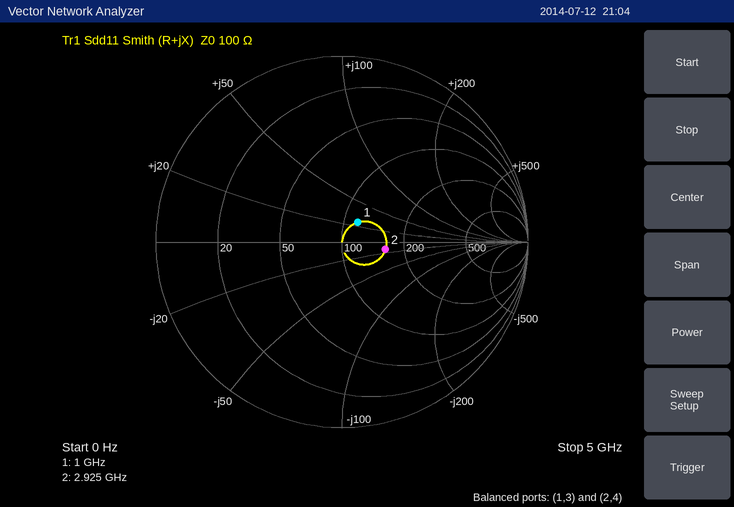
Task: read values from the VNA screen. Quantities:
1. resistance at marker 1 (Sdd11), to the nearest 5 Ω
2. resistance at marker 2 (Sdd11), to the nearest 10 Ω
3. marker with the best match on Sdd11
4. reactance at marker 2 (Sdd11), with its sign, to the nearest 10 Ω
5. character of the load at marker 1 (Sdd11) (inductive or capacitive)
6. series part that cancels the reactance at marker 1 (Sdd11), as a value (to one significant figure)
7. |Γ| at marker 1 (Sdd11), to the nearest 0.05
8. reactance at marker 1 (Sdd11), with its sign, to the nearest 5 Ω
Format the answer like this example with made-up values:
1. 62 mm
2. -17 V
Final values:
1. 115 Ω
2. 160 Ω
3. marker 1
4. -10 Ω
5. inductive
6. 6 pF
7. 0.15
8. +25 Ω
